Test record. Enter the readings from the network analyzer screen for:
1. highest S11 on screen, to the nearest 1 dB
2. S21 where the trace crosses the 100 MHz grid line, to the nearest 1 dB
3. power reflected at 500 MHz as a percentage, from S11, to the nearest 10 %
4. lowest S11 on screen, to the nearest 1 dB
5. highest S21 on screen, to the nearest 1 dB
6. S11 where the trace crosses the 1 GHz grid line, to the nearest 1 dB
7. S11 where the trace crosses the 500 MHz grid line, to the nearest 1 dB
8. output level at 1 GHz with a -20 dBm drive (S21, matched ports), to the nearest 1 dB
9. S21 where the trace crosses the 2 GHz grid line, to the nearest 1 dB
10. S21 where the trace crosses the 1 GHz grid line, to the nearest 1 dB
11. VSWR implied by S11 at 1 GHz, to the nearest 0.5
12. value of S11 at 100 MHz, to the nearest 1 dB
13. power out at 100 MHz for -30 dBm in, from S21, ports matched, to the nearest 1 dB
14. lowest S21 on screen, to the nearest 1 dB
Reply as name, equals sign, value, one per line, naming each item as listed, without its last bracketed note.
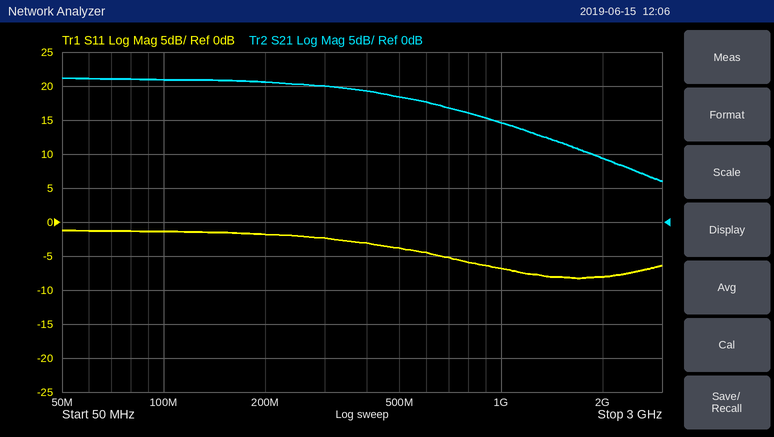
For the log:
highest S11 on screen, to the nearest 1 dB = -1 dB
S21 where the trace crosses the 100 MHz grid line, to the nearest 1 dB = 21 dB
power reflected at 500 MHz as a percentage, from S11, to the nearest 10 % = 40 %
lowest S11 on screen, to the nearest 1 dB = -8 dB
highest S21 on screen, to the nearest 1 dB = 21 dB
S11 where the trace crosses the 1 GHz grid line, to the nearest 1 dB = -7 dB
S11 where the trace crosses the 500 MHz grid line, to the nearest 1 dB = -4 dB
output level at 1 GHz with a -20 dBm drive (S21, matched ports), to the nearest 1 dB = -5 dBm
S21 where the trace crosses the 2 GHz grid line, to the nearest 1 dB = 9 dB
S21 where the trace crosses the 1 GHz grid line, to the nearest 1 dB = 15 dB
VSWR implied by S11 at 1 GHz, to the nearest 0.5 = 2.5
value of S11 at 100 MHz, to the nearest 1 dB = -1 dB
power out at 100 MHz for -30 dBm in, from S21, ports matched, to the nearest 1 dB = -9 dBm
lowest S21 on screen, to the nearest 1 dB = 6 dB
